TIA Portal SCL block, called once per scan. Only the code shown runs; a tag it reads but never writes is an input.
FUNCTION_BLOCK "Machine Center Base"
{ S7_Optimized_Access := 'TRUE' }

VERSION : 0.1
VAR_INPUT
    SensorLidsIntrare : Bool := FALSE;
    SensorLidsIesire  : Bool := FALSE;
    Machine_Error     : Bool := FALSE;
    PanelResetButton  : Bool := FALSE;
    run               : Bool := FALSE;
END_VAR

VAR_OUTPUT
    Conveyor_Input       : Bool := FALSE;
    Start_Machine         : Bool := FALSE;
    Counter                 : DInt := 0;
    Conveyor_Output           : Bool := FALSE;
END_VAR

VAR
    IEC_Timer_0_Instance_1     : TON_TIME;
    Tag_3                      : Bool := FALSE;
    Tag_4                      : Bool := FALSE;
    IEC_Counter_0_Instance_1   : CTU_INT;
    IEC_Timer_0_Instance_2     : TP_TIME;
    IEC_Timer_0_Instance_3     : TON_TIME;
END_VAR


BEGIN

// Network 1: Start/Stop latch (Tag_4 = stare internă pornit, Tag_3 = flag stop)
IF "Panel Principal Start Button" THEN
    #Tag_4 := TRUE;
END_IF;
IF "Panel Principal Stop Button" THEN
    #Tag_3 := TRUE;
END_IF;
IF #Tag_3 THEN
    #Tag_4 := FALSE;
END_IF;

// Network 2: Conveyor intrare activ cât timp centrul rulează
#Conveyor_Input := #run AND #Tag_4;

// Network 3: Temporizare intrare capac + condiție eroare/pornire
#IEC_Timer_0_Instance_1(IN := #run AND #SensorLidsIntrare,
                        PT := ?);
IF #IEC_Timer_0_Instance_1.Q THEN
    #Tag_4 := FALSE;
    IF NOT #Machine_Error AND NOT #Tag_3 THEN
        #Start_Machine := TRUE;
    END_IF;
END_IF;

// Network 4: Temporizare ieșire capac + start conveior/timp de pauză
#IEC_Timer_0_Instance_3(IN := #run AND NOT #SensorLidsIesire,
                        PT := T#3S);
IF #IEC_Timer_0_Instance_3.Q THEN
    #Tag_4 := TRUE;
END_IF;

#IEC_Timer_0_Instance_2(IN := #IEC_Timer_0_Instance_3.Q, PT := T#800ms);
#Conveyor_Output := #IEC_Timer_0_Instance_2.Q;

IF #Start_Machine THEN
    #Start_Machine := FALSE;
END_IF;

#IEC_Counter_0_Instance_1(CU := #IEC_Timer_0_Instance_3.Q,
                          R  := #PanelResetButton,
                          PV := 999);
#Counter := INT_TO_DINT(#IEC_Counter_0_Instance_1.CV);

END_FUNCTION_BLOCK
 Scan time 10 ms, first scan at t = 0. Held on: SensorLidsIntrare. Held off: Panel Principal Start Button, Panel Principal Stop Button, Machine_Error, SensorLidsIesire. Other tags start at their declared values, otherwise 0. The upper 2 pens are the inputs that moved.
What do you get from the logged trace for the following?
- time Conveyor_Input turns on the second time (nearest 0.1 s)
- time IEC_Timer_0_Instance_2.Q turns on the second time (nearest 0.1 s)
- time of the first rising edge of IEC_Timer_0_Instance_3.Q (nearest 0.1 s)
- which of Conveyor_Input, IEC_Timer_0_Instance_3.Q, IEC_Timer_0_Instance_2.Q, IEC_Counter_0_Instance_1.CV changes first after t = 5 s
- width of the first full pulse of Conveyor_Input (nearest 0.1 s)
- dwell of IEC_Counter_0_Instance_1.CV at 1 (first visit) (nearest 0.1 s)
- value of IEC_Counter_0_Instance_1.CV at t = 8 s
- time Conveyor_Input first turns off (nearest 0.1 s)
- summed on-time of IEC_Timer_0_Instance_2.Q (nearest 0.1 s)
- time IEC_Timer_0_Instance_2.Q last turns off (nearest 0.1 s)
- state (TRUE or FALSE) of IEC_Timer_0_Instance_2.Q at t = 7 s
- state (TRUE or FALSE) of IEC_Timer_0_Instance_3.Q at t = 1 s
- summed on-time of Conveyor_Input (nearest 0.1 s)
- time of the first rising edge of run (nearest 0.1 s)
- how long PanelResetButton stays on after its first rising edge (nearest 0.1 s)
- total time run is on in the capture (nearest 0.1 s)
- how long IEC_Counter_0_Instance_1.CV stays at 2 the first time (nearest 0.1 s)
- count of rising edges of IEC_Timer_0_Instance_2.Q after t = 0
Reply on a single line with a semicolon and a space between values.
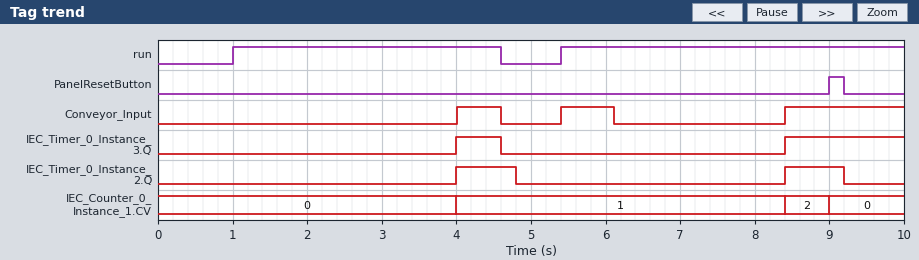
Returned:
5.4 s; 8.4 s; 4.0 s; Conveyor_Input; 0.6 s; 4.4 s; 1; 4.6 s; 1.6 s; 9.2 s; FALSE; FALSE; 2.9 s; 1.0 s; 0.2 s; 8.2 s; 0.6 s; 2
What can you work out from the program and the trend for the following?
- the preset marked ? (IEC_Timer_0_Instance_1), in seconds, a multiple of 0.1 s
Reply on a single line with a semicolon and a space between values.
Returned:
0.7 s
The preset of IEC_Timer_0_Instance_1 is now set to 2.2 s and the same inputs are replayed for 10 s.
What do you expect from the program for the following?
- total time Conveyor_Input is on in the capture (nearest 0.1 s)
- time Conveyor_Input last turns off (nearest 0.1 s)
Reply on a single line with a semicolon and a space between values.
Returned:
4.4 s; 7.6 s
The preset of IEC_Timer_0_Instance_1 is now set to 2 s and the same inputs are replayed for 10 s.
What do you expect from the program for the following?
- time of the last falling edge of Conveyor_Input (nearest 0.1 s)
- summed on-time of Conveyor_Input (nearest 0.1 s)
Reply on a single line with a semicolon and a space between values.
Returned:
7.4 s; 4.2 s
